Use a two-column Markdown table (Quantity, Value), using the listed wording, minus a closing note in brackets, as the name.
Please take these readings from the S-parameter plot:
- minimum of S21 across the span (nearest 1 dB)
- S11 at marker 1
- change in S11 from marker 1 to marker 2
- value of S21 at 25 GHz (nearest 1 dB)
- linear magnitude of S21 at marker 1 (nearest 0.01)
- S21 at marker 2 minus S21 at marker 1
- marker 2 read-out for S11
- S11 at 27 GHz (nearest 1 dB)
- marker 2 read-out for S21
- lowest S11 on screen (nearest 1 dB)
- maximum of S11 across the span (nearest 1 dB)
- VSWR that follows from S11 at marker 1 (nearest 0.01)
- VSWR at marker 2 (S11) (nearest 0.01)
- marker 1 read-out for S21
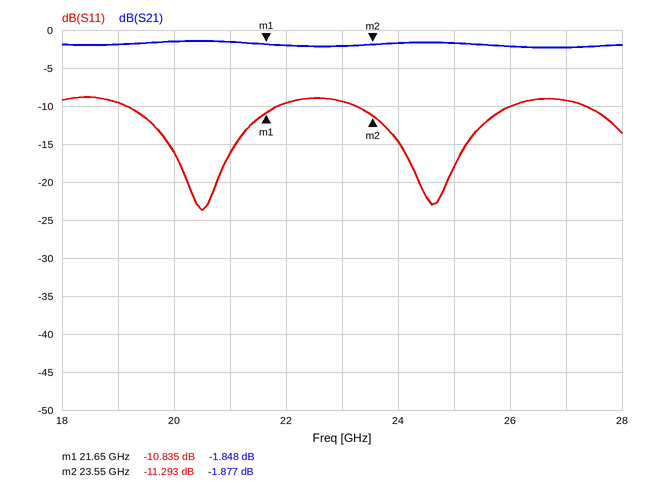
| Quantity | Value |
|---|---|
| minimum of S21 across the span | -2 dB |
| S11 at marker 1 | -10.835 dB |
| change in S11 from marker 1 to marker 2 | -0.458 dB |
| value of S21 at 25 GHz | -2 dB |
| linear magnitude of S21 at marker 1 | 0.81 |
| S21 at marker 2 minus S21 at marker 1 | -0.029 dB |
| marker 2 read-out for S11 | -11.293 dB |
| S11 at 27 GHz | -9 dB |
| marker 2 read-out for S21 | -1.877 dB |
| lowest S11 on screen | -24 dB |
| maximum of S11 across the span | -9 dB |
| VSWR that follows from S11 at marker 1 | 1.81 |
| VSWR at marker 2 (S11) | 1.75 |
| marker 1 read-out for S21 | -1.848 dB |
